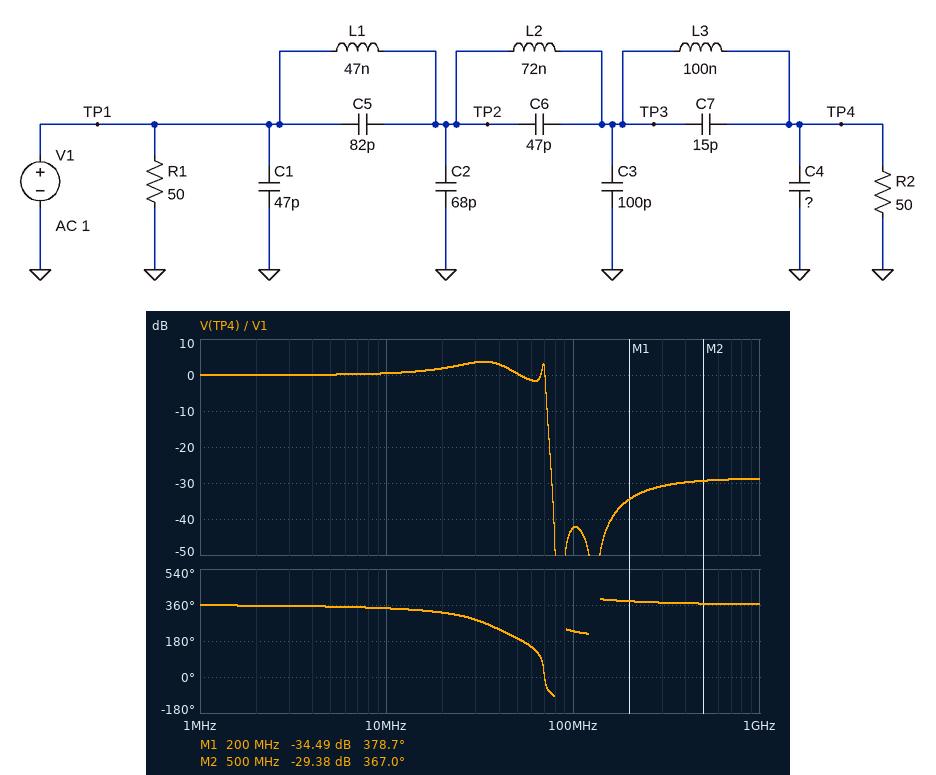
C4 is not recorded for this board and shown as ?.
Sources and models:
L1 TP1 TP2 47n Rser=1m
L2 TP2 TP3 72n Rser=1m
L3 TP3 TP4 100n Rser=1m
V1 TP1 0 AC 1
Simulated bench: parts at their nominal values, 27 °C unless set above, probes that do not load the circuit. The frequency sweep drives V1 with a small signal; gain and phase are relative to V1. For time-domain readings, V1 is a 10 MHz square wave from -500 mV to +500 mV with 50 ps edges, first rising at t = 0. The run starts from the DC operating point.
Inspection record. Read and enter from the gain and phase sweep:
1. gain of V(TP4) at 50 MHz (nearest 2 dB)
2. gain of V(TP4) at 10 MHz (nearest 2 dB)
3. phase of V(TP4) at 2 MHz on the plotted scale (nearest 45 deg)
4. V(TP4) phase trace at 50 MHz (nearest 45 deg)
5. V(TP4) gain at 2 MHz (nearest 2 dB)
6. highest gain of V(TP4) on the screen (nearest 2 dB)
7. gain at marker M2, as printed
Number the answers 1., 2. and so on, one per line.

1. 0 dB
2. 0 dB
3. 360 deg
4. 180 deg
5. 0 dB
6. 4 dB
7. -29.38 dB
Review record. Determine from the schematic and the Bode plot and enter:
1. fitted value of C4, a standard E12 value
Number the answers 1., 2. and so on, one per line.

1. 39 pF
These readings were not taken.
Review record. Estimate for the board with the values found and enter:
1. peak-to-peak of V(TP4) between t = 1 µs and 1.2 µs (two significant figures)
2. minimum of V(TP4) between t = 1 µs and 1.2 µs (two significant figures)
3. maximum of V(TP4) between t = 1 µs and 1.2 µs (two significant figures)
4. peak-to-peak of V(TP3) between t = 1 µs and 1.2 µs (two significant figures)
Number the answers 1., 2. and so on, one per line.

1. 1.9 V
2. -960 mV
3. 960 mV
4. 1.9 V
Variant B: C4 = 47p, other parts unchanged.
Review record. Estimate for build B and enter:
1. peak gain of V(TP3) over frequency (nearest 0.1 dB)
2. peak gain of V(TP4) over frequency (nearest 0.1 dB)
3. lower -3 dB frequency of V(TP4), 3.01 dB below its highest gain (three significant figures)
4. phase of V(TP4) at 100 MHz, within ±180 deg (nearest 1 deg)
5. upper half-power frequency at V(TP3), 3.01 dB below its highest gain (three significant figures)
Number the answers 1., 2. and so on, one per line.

1. 4.3 dB
2. 3.7 dB
3. 11.4 MHz
4. -138 deg
5. 70.7 MHz
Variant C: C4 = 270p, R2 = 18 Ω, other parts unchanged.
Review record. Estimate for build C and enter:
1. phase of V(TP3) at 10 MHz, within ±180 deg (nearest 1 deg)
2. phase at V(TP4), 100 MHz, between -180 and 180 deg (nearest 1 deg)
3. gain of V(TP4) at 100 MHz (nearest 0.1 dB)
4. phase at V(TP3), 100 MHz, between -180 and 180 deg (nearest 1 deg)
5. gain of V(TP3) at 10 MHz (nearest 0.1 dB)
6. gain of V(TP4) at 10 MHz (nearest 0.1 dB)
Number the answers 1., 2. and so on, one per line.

1. -25 deg
2. -161 deg
3. -58.7 dB
4. 0 deg
5. -0.6 dB
6. -0.3 dB
